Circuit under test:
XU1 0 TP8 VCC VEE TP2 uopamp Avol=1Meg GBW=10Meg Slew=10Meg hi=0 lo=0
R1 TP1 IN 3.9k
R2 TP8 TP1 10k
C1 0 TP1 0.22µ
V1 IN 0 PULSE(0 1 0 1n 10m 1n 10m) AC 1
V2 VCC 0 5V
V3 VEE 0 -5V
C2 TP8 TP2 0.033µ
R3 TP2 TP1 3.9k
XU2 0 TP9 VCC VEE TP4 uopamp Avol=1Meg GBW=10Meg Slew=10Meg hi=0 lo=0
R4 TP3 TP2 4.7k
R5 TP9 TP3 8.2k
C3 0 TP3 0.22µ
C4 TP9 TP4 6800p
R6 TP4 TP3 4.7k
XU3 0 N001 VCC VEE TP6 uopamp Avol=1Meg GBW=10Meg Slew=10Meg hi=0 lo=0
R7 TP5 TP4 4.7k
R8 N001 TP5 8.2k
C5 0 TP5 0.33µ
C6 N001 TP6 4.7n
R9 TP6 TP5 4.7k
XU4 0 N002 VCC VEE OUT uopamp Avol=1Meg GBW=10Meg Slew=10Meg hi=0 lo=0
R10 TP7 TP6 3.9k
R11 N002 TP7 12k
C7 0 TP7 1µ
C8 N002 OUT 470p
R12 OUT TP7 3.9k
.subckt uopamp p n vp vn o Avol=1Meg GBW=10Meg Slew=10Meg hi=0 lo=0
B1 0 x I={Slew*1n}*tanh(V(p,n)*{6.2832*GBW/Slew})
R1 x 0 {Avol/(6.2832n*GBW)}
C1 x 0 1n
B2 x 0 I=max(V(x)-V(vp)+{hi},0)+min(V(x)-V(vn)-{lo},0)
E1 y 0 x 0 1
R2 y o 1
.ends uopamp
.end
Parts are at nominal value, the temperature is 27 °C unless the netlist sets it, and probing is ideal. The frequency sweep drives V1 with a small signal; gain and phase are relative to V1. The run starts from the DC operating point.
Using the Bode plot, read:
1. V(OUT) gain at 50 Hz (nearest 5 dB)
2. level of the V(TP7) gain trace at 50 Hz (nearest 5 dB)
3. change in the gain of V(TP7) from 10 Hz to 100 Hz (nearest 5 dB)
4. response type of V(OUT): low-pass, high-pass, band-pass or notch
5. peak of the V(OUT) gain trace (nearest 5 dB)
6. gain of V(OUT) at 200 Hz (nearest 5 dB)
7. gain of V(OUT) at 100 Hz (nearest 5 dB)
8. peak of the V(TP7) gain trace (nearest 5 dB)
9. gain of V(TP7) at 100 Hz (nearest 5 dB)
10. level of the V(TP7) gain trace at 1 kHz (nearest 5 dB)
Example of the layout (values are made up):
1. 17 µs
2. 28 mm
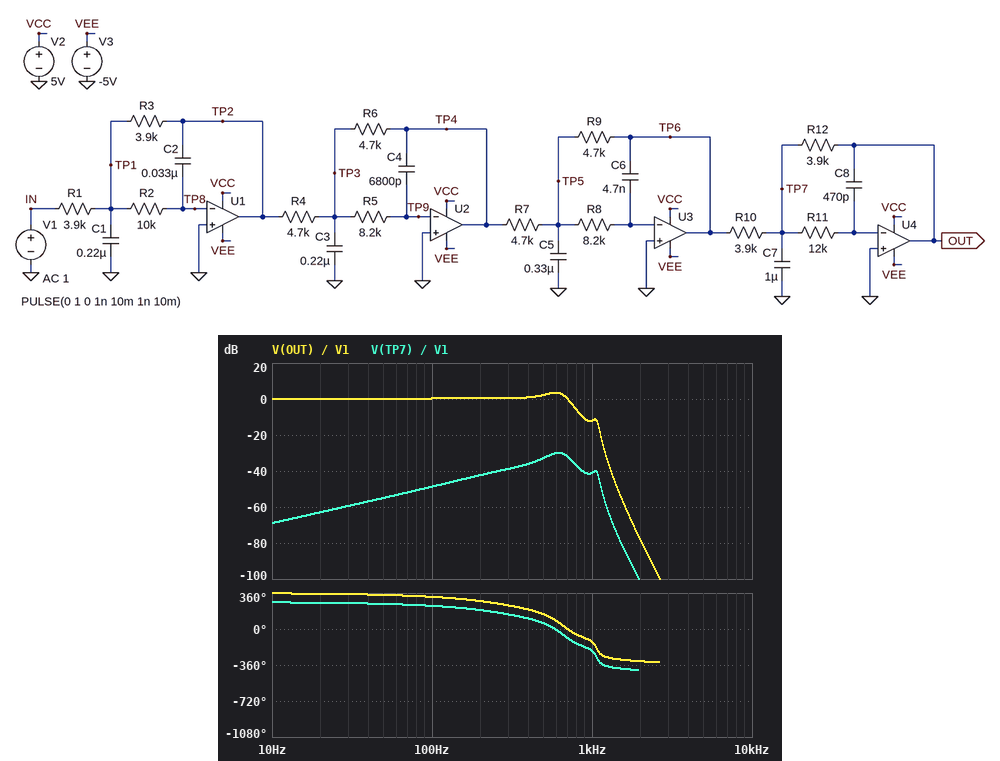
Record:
1. 0 dB
2. -55 dB
3. 20 dB
4. low-pass
5. 5 dB
6. 0 dB
7. 0 dB
8. -30 dB
9. -50 dB
10. -40 dB
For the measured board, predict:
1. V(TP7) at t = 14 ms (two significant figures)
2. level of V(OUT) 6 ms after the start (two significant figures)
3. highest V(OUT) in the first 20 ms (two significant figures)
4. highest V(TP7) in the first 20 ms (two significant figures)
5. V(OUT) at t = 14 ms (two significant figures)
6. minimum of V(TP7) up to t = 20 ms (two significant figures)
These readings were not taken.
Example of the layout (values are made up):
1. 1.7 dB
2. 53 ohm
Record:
1. 1.7 mV
2. 490 mV
3. 1.2 V
4. 5.1 mV
5. 670 mV
6. -10 mV
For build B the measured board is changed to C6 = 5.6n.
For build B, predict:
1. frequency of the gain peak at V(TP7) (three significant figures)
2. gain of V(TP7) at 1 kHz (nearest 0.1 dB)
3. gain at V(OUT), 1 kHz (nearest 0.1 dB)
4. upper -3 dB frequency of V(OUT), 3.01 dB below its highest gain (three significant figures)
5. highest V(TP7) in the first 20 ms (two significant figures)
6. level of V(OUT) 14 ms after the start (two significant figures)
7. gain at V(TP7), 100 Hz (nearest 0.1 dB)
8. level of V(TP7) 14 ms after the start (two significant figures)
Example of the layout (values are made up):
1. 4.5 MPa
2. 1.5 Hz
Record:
1. 575 Hz
2. -43.5 dB
3. -14.5 dB
4. 652 Hz
5. 4.6 mV
6. 720 mV
7. -48.7 dB
8. 2.0 mV
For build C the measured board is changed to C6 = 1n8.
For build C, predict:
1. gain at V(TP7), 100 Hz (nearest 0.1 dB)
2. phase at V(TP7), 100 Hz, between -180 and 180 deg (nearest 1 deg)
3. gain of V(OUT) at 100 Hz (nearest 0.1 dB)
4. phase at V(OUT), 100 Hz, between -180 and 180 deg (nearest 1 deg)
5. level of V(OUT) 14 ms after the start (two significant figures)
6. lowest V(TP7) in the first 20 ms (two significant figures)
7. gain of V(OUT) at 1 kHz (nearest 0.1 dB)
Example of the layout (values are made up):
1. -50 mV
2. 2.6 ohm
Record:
1. -48.8 dB
2. -126 deg
3. 0.2 dB
4. -36 deg
5. 640 mV
6. -11 mV
7. 3.1 dB
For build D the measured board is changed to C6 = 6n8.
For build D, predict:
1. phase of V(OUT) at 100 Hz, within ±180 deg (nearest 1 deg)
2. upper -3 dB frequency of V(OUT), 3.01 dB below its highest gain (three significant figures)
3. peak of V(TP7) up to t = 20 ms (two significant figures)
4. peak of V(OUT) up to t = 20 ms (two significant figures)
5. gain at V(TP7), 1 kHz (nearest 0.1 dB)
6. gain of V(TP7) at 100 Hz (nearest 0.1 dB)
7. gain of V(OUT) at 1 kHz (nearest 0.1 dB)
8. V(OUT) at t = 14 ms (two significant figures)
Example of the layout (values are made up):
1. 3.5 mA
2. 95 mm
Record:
1. -40 deg
2. 604 Hz
3. 4.2 mV
4. 1.2 V
5. -45.9 dB
6. -48.6 dB
7. -16.9 dB
8. 760 mV
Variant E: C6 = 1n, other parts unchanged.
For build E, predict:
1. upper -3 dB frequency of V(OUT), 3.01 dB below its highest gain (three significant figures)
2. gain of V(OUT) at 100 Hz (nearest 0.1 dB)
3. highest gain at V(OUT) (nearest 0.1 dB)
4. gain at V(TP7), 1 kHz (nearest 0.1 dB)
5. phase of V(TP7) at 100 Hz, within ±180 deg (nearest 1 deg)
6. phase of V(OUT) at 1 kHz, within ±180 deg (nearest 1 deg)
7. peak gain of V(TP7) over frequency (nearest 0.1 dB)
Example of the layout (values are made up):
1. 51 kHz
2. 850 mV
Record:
1. 1.11 kHz
2. 0.1 dB
3. 0.4 dB
4. -31.9 dB
5. -126 deg
6. 14 deg
7. -28.0 dB
